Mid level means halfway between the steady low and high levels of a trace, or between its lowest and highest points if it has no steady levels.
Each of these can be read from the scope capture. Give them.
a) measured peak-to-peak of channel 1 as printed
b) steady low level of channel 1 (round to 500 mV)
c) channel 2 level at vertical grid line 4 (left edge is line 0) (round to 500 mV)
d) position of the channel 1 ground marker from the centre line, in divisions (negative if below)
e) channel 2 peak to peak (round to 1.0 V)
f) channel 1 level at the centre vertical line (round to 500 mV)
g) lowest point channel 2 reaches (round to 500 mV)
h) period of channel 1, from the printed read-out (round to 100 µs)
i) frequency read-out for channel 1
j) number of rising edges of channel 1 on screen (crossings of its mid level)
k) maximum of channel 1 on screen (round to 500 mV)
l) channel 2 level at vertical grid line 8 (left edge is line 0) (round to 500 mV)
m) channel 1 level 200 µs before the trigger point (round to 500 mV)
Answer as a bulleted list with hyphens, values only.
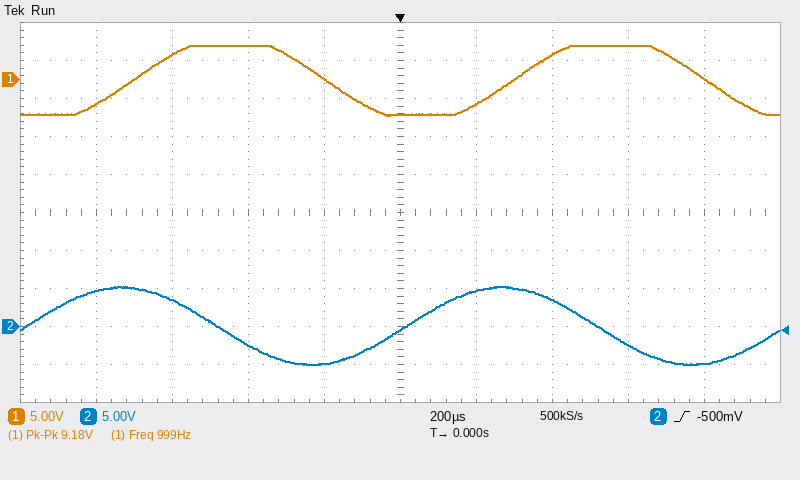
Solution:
- 9.18 V
- -4.5 V
- -5.0 V
- +3.5 div
- 10.0 V
- -4.5 V
- -5.0 V
- 1.0 ms
- 999 Hz
- 2
- 4.5 V
- -2.5 V
- 0.0 V
